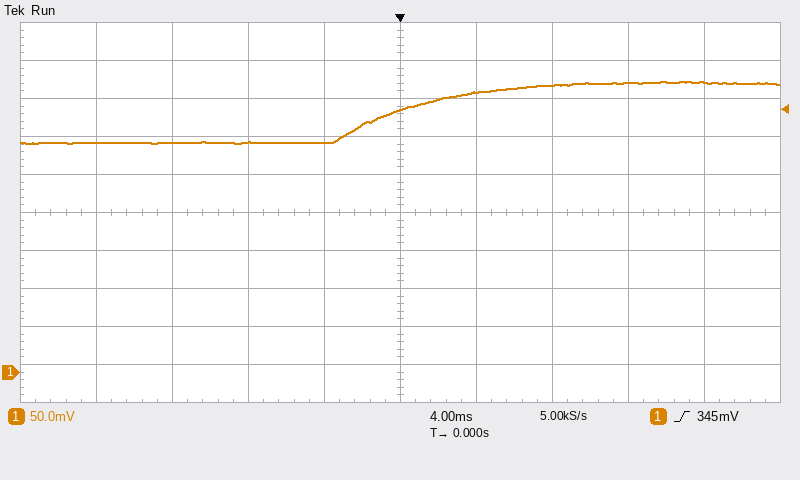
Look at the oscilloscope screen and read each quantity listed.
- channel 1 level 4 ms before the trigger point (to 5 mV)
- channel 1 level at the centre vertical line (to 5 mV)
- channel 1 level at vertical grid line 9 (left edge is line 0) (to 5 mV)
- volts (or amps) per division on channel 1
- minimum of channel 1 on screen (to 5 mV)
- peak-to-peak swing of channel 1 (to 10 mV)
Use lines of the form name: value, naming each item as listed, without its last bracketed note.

channel 1 level 4 ms before the trigger point: 300 mV
channel 1 level at the centre vertical line: 345 mV
channel 1 level at vertical grid line 9 (left edge is line 0): 380 mV
volts (or amps) per division on channel 1: 50 mV
minimum of channel 1 on screen: 300 mV
peak-to-peak swing of channel 1: 80 mV
